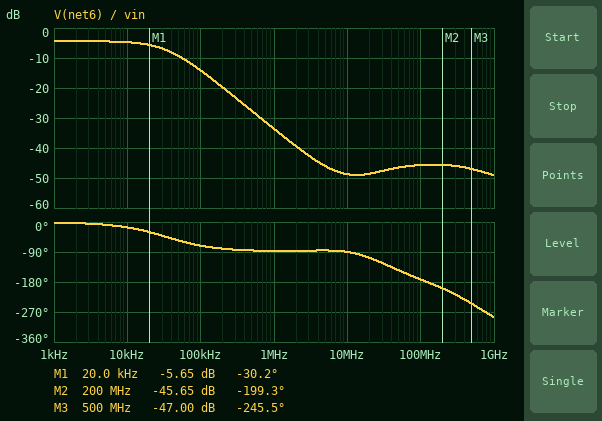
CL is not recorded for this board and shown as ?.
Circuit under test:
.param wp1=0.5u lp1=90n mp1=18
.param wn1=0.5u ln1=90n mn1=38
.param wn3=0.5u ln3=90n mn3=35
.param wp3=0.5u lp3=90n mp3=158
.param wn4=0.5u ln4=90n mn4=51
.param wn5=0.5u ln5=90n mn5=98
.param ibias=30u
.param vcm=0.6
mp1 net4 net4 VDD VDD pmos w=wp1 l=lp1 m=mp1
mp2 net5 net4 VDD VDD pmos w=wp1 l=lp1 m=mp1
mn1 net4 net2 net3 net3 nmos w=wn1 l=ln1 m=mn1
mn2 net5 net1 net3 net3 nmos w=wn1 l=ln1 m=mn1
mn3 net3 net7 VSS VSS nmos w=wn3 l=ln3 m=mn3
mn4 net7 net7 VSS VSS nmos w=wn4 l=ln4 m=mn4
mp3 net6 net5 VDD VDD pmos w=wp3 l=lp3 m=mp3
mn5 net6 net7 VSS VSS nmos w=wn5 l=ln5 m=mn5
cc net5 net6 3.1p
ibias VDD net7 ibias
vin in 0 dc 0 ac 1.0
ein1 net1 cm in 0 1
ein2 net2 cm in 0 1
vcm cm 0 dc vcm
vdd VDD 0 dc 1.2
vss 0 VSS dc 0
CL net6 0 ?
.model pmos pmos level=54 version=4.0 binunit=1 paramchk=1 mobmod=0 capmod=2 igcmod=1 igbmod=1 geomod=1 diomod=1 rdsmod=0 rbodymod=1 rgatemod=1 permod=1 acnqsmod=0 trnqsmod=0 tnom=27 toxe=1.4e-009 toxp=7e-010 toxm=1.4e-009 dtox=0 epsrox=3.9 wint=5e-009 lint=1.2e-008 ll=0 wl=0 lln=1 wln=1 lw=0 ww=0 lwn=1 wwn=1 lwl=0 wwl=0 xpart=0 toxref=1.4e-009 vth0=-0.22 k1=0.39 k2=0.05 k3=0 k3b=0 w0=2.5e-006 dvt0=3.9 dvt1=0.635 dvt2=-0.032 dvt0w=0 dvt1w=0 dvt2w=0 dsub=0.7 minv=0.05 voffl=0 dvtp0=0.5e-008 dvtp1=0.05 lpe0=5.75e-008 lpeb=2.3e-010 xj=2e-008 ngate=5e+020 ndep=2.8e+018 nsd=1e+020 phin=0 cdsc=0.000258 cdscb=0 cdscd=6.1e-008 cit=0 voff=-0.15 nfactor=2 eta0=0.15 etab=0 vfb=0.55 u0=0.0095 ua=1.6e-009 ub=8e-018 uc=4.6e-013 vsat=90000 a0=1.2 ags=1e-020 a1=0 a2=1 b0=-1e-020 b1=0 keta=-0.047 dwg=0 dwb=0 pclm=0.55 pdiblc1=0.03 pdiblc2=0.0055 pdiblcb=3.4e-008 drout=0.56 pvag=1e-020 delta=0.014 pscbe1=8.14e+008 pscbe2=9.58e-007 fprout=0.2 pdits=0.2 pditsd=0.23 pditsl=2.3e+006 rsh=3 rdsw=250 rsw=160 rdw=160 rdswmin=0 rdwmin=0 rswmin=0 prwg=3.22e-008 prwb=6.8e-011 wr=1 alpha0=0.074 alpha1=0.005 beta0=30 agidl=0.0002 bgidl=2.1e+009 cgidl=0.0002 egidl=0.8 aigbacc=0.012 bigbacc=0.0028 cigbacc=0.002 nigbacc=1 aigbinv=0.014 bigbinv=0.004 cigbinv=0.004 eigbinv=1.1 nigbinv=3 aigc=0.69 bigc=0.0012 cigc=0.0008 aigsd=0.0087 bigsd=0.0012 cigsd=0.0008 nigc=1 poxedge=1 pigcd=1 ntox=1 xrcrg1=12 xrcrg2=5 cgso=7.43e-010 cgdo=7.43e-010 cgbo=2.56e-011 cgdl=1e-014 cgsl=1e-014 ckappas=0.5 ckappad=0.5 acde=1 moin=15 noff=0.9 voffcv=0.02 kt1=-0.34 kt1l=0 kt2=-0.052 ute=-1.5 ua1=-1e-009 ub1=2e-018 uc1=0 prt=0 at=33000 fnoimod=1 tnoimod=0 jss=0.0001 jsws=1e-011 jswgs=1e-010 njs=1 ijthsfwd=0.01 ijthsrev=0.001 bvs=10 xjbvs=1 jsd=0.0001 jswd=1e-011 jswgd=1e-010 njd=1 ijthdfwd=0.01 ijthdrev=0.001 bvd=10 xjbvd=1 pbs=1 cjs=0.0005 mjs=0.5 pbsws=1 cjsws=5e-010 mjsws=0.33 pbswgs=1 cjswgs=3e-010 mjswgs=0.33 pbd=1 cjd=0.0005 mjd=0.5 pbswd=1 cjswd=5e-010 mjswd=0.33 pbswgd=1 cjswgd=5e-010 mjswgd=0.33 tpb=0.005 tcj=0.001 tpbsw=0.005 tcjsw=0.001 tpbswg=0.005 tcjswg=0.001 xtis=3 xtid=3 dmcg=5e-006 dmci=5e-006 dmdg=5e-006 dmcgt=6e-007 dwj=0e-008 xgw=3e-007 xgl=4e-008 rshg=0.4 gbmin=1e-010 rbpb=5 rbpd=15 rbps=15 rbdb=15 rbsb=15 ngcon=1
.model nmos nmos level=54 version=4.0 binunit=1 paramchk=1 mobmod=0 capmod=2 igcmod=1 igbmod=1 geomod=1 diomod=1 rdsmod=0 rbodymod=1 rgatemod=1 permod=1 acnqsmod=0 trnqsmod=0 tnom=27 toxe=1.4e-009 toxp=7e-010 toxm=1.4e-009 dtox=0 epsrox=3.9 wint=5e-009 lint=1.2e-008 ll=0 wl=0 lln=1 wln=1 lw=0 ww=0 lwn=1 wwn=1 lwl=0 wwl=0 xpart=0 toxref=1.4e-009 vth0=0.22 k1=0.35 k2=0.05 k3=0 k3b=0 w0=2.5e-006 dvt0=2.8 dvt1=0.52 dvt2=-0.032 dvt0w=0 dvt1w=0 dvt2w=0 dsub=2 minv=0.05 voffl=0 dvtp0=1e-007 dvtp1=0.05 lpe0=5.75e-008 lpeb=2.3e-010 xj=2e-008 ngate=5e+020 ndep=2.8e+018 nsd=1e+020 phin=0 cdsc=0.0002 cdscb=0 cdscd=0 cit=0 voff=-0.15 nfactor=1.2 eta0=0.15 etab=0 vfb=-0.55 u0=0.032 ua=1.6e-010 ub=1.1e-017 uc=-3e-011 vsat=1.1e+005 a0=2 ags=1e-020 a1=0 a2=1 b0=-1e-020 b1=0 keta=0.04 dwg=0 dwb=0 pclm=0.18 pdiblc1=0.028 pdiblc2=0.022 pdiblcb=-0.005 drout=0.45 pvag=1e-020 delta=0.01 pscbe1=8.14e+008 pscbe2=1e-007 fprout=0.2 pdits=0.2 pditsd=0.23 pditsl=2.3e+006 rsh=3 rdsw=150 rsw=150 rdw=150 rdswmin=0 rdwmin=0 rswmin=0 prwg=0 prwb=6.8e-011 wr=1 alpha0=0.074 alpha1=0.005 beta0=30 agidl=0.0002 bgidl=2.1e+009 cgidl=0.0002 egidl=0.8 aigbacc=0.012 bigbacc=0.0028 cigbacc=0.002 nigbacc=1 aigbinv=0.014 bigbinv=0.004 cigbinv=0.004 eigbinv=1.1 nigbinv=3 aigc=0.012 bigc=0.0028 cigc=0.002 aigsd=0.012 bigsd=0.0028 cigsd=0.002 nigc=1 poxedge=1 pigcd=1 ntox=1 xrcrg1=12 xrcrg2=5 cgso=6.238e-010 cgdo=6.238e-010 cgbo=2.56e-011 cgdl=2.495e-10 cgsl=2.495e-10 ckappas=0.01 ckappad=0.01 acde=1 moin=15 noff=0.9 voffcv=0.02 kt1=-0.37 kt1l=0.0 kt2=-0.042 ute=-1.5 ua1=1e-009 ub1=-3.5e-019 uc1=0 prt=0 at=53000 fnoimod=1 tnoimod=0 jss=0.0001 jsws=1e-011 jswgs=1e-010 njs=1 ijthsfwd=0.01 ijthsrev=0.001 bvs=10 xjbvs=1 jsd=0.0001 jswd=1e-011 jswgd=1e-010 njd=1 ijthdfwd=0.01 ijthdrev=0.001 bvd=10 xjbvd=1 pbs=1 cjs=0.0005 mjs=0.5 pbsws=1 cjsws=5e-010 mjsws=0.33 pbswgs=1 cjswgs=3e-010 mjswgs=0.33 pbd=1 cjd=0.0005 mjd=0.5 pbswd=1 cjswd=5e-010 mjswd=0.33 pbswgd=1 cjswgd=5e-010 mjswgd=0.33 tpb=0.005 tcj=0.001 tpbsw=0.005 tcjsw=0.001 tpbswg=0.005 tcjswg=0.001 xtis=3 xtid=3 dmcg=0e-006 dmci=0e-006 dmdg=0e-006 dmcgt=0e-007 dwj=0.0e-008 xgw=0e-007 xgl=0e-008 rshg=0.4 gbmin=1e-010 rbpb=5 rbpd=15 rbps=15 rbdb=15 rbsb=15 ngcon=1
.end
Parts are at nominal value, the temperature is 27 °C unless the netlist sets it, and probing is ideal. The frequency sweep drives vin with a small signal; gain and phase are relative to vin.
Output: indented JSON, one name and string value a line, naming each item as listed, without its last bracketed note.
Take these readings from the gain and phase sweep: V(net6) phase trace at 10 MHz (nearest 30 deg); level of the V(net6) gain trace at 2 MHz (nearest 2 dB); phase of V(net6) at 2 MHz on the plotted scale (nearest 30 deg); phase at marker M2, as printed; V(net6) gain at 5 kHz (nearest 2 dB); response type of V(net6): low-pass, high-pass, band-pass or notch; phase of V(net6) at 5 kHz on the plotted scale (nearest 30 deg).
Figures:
{
  "V(net6) phase trace at 10 MHz": "-90 deg",
  "level of the V(net6) gain trace at 2 MHz": "-40 dB",
  "phase of V(net6) at 2 MHz on the plotted scale": "-90 deg",
  "phase at marker M2, as printed": "-199.3 deg",
  "V(net6) gain at 5 kHz": "-4 dB",
  "response type of V(net6): low-pass, high-pass, band-pass or notch": "low-pass",
  "phase of V(net6) at 5 kHz on the plotted scale": "0 deg"
}
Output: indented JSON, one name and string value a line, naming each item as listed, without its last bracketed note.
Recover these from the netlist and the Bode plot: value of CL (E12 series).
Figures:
{
  "value of CL": "6.8 pF"
}
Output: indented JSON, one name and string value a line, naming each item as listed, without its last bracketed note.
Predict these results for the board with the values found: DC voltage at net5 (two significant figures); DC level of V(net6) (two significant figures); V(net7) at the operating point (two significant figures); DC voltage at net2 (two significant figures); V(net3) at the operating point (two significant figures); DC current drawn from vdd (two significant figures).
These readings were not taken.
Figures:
{
  "DC voltage at net5": "870 mV",
  "DC level of V(net6)": "940 mV",
  "V(net7) at the operating point": "300 mV",
  "DC voltage at net2": "600 mV",
  "V(net3) at the operating point": "340 mV",
  "DC current drawn from vdd": "140 µA"
}
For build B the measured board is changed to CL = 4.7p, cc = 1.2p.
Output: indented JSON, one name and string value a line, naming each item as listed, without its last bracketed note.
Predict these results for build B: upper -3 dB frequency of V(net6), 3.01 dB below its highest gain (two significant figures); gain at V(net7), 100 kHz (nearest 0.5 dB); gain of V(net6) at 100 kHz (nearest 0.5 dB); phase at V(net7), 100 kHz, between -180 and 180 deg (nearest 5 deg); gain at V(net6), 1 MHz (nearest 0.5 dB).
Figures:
{
  "upper -3 dB frequency of V(net6), 3.01 dB below its highest gain": "84 kHz",
  "gain at V(net7), 100 kHz": "-45.0 dB",
  "gain of V(net6) at 100 kHz": "-8.0 dB",
  "phase at V(net7), 100 kHz, between -180 and 180 deg": "-50 deg",
  "gain at V(net6), 1 MHz": "-26.0 dB"
}
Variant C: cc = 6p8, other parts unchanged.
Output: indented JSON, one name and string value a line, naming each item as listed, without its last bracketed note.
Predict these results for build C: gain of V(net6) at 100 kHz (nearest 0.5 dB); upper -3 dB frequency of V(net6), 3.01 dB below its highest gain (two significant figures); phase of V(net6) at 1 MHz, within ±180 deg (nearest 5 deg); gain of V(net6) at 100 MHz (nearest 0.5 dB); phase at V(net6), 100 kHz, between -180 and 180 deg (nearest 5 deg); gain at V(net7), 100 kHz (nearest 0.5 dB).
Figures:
{
  "gain of V(net6) at 100 kHz": "-20.5 dB",
  "upper -3 dB frequency of V(net6), 3.01 dB below its highest gain": "16 kHz",
  "phase of V(net6) at 1 MHz, within ±180 deg": "-90 deg",
  "gain of V(net6) at 100 MHz": "-46.0 dB",
  "phase at V(net6), 100 kHz, between -180 and 180 deg": "-80 deg",
  "gain at V(net7), 100 kHz": "-57.5 dB"
}
